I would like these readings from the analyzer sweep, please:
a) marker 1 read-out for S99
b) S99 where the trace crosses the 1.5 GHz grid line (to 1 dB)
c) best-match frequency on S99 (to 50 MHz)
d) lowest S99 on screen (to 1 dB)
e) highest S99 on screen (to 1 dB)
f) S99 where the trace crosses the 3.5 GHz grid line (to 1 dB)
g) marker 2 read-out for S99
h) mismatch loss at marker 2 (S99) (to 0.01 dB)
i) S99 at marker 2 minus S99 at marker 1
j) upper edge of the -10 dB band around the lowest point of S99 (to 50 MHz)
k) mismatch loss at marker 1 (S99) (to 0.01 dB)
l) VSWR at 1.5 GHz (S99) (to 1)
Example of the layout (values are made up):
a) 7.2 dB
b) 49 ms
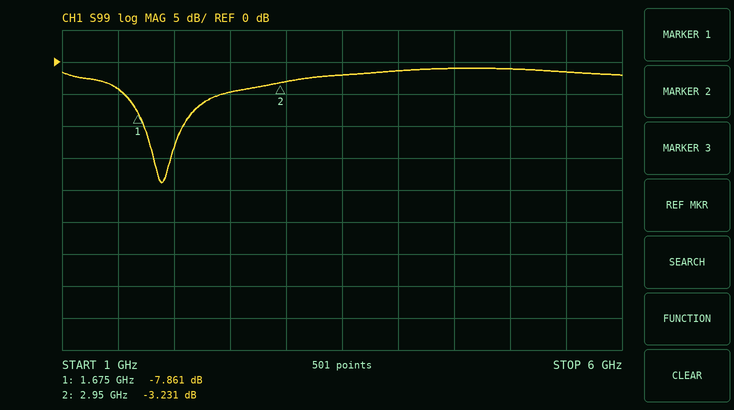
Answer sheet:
a) -7.861 dB
b) -4 dB
c) 1.90 GHz
d) -19 dB
e) -1 dB
f) -2 dB
g) -3.231 dB
h) 2.80 dB
i) 4.630 dB
j) 2.10 GHz
k) 0.78 dB
l) 4
